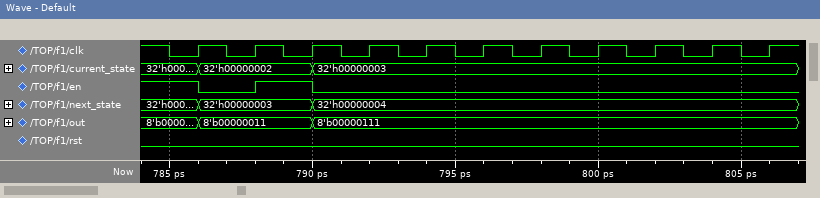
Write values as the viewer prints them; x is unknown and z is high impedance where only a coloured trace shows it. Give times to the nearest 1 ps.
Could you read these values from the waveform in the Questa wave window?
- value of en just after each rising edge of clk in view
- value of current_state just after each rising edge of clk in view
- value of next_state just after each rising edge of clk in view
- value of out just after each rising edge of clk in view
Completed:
0 1 0 0 0 0 0 0 0 0 0
32'h00000002, 32'h00000002, 32'h00000003, 32'h00000003, 32'h00000003, 32'h00000003, 32'h00000003, 32'h00000003, 32'h00000003, 32'h00000003, 32'h00000003
32'h00000003, 32'h00000003, 32'h00000004, 32'h00000004, 32'h00000004, 32'h00000004, 32'h00000004, 32'h00000004, 32'h00000004, 32'h00000004, 32'h00000004
8'b00000011, 8'b00000011, 8'b00000111, 8'b00000111, 8'b00000111, 8'b00000111, 8'b00000111, 8'b00000111, 8'b00000111, 8'b00000111, 8'b00000111
